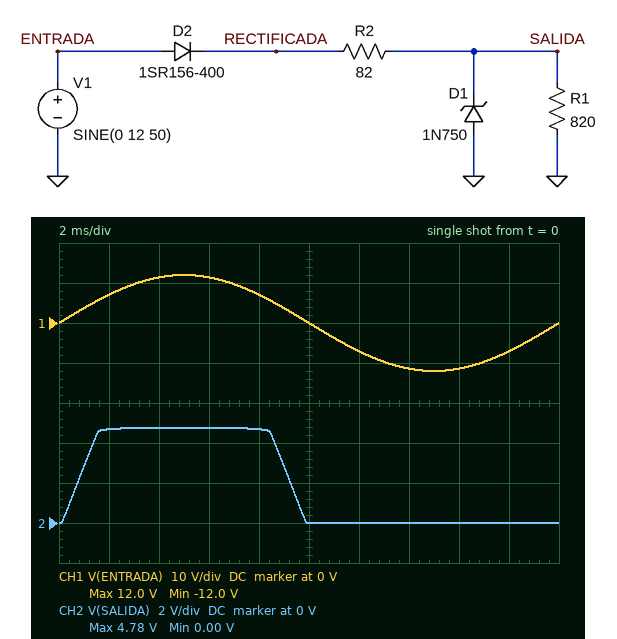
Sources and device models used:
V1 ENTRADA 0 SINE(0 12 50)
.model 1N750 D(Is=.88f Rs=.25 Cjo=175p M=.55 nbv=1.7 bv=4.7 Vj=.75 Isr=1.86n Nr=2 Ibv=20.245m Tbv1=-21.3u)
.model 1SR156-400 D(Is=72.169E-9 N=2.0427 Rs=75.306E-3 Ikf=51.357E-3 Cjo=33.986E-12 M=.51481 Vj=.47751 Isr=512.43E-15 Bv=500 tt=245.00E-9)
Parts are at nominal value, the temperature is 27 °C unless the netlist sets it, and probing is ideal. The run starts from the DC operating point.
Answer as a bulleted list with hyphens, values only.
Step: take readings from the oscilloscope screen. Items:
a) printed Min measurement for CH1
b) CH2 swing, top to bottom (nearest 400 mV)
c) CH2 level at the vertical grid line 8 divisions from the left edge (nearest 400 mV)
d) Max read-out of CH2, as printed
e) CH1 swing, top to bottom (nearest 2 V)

- -12.0 V
- 4.8 V
- 0 V
- 4.78 V
- 24 V
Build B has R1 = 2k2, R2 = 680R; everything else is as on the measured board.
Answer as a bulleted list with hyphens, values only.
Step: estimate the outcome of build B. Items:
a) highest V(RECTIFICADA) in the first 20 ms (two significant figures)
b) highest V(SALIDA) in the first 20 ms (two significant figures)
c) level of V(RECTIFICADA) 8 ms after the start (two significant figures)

- 11 V
- 4.7 V
- 6.5 V
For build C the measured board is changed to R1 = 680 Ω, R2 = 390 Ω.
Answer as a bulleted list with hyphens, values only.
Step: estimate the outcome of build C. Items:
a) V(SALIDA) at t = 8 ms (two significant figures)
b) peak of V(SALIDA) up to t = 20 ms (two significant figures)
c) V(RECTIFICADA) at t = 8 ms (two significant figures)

- 4.1 V
- 4.7 V
- 6.4 V
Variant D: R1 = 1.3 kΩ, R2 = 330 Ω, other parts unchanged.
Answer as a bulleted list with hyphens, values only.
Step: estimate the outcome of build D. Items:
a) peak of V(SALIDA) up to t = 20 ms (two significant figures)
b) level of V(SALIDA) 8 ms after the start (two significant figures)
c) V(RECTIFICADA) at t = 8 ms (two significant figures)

- 4.7 V
- 4.6 V
- 6.4 V
